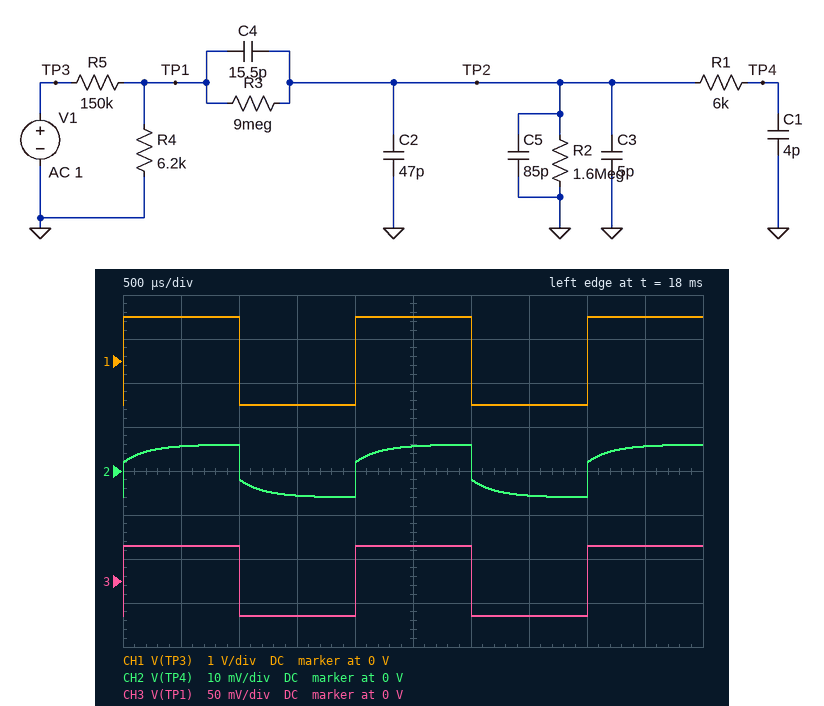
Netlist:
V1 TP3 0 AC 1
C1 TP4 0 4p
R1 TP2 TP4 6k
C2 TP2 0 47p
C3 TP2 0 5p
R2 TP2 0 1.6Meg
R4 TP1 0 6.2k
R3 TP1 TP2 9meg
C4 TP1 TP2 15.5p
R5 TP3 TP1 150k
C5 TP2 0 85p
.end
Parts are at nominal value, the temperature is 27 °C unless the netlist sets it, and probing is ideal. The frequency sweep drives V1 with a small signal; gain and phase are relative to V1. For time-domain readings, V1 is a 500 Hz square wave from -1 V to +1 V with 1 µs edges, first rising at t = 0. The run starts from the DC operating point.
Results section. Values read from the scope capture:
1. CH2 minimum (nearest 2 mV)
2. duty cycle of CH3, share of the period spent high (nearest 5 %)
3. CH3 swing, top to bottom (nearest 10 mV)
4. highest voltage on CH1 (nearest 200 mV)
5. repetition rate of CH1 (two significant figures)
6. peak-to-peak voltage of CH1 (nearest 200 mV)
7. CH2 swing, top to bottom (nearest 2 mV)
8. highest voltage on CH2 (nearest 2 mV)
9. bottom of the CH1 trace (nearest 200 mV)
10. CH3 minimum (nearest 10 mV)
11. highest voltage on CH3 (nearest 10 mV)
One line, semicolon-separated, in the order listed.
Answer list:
-6 mV; 50 %; 80 mV; 1.0 V; 500 Hz; 2.0 V; 12 mV; 6 mV; -1.0 V; -40 mV; 40 mV
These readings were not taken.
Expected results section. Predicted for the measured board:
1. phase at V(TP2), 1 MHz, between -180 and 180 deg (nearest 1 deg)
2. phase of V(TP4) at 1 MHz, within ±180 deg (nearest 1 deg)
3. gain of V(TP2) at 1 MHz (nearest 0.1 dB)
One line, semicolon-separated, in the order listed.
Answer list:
-27 deg; -36 deg; -49.2 dB
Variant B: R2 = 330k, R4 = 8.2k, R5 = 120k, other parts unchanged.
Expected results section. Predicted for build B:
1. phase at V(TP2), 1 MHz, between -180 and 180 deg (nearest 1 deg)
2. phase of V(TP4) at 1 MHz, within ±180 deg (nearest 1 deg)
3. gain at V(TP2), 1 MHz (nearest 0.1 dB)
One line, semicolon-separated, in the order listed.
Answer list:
-34 deg; -42 deg; -45.6 dB
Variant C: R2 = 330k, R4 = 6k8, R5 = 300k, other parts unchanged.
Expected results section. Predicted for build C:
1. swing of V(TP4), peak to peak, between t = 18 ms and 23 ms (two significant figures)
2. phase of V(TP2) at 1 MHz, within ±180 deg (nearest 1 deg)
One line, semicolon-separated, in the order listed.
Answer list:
7.1 mV; -30 deg
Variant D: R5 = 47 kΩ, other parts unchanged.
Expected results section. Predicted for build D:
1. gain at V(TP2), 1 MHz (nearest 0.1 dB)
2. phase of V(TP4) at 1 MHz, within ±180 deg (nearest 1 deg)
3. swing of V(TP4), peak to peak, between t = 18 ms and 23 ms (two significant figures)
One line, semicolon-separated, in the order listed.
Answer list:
-39.7 dB; -34 deg; 35 mV
